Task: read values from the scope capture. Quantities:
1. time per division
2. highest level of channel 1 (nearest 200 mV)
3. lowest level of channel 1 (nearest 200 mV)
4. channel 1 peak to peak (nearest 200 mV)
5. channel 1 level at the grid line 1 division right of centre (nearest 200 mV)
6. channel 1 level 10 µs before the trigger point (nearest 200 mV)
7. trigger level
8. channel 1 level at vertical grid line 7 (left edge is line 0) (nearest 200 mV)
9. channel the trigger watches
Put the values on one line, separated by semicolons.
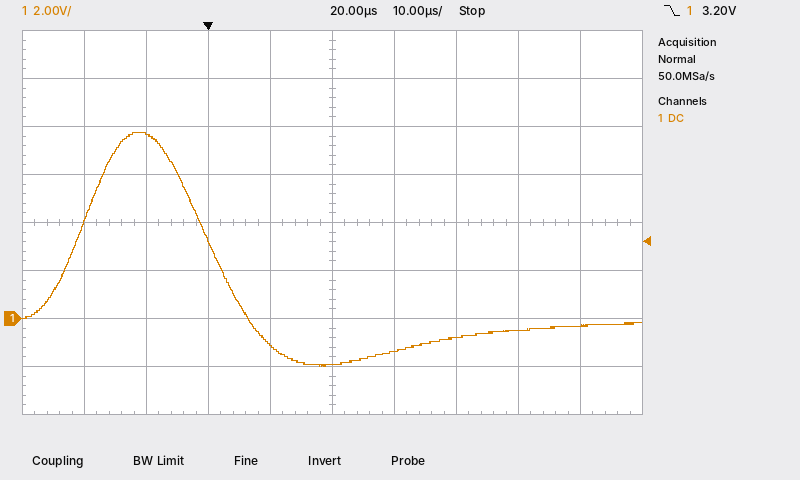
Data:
10 µs; 7.8 V; -2.0 V; 9.8 V; -1.4 V; 7.6 V; 3.20 V; -800 mV; channel 1
